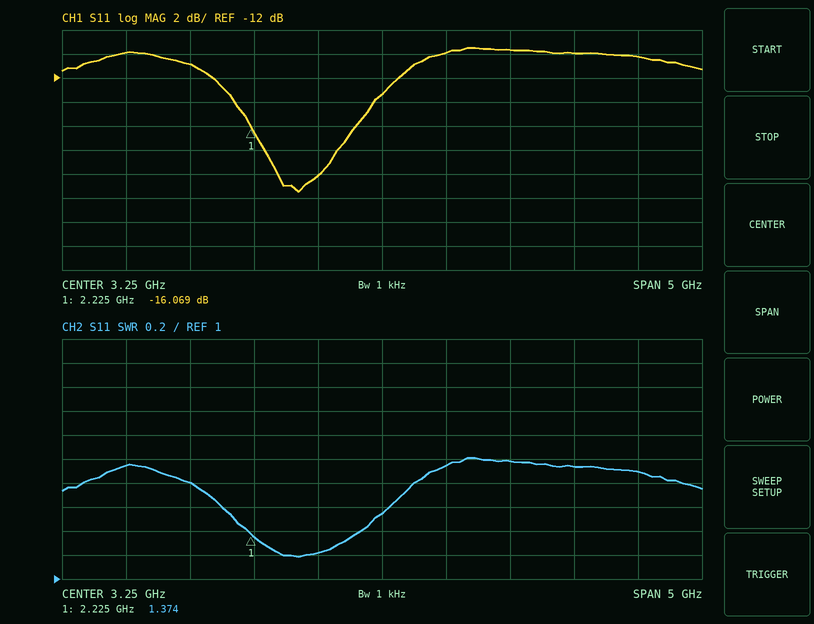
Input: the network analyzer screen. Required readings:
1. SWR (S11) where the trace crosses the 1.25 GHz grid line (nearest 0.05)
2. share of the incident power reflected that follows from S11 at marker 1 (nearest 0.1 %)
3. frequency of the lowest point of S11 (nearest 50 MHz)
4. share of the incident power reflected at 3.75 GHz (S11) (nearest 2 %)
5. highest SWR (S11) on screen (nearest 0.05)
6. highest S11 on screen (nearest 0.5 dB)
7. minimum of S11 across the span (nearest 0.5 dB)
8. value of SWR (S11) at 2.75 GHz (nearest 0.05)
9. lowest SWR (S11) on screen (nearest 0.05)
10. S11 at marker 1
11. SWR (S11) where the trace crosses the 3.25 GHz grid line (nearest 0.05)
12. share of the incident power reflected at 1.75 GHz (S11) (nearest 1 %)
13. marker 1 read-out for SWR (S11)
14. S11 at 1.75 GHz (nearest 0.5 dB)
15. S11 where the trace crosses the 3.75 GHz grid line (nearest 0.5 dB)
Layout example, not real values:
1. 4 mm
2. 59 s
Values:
1. 1.95
2. 2.5 %
3. 2.60 GHz
4. 10 %
5. 2.00
6. -9.5 dB
7. -21.5 dB
8. 1.20
9. 1.20
10. -16.069 dB
11. 1.55
12. 8 %
13. 1.374
14. -11.0 dB
15. -10.0 dB
